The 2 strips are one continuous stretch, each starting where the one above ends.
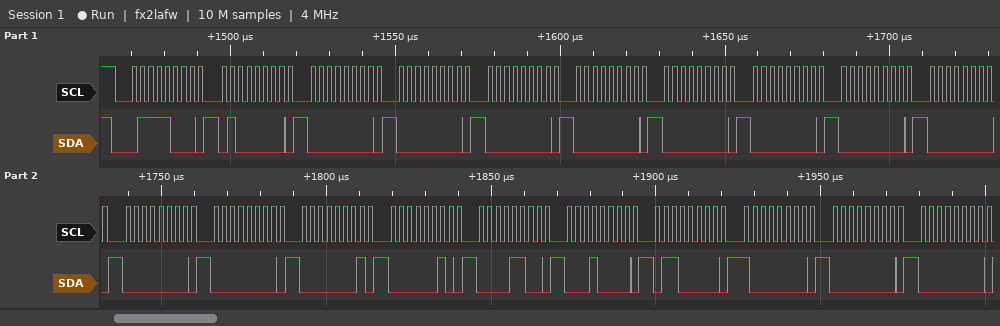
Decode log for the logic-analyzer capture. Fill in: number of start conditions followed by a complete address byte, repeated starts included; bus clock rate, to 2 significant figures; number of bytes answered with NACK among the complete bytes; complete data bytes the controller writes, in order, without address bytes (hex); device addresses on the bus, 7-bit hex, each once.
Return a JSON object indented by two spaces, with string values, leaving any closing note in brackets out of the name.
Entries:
{
  "number of start conditions followed by a complete address byte, repeated starts included": "1",
  "bus clock rate, to 2 significant figures": "400 kHz",
  "number of bytes answered with NACK among the complete bytes": "0",
  "complete data bytes the controller writes, in order, without address bytes": "40 00 00 00 00 00 00 00 00 00 00 01 02 0C 10 60 80 00 00",
  "device addresses on the bus, 7-bit hex, each once": "0x3C"
}
